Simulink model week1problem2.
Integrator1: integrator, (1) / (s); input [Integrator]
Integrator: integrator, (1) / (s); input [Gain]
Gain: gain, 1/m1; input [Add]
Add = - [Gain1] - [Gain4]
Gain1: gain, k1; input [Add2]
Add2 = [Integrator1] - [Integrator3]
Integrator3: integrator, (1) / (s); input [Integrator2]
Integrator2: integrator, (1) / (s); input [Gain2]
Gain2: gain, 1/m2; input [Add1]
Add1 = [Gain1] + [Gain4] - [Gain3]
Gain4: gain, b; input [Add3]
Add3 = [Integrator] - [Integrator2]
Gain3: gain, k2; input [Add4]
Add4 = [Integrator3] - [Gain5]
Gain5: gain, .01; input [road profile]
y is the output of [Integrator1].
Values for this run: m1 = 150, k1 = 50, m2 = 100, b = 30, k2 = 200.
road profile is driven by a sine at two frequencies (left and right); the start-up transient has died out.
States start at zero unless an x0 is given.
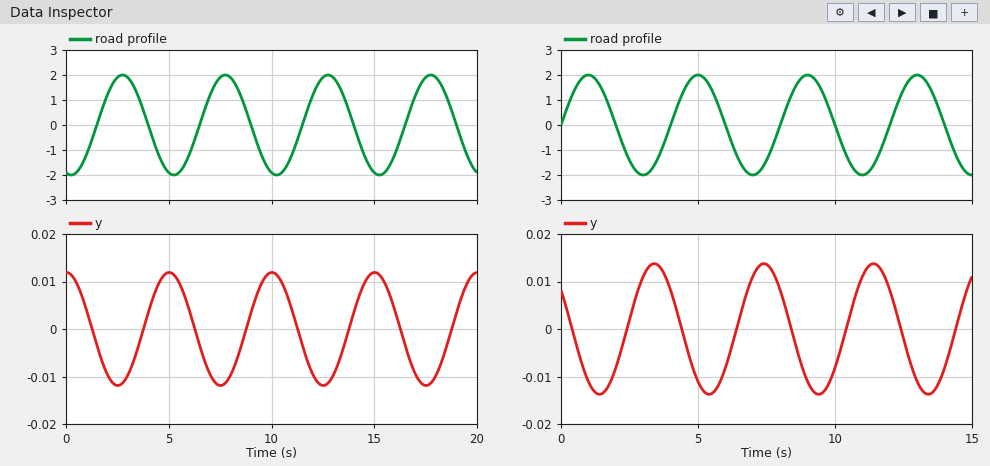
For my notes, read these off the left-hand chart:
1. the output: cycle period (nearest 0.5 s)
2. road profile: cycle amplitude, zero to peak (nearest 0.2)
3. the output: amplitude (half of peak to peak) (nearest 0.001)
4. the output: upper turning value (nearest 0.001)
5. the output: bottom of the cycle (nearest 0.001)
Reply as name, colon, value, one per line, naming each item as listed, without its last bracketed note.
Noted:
the output: cycle period: 5.0 s
road profile: cycle amplitude, zero to peak: 2.0
the output: amplitude (half of peak to peak): 0.012
the output: upper turning value: 0.012
the output: bottom of the cycle: -0.012
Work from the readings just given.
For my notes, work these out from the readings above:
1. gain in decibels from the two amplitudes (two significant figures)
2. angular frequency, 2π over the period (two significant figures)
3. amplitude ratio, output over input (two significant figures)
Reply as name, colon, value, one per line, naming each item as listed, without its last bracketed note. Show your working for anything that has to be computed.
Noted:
gain in decibels from the two amplitudes: 20 log10(0.012 / 2) = -44 dB
angular frequency, 2π over the period: 2π / 5 = 1.3 rad/s
amplitude ratio, output over input: 0.012 / 2 = 0.0060
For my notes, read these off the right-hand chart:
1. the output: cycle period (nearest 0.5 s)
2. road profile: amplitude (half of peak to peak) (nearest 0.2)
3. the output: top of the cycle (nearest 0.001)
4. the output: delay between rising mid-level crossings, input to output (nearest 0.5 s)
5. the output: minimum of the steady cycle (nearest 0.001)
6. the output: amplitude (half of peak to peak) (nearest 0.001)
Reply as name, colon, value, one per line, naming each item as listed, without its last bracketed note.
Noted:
the output: cycle period: 4.0 s
road profile: amplitude (half of peak to peak): 2.0
the output: top of the cycle: 0.014
the output: delay between rising mid-level crossings, input to output: 2.5 s
the output: minimum of the steady cycle: -0.014
the output: amplitude (half of peak to peak): 0.014
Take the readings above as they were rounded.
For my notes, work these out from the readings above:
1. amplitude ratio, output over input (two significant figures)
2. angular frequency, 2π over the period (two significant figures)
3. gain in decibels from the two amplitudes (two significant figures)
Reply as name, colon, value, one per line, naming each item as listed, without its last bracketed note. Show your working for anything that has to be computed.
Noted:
amplitude ratio, output over input: 0.014 / 2 = 0.0070
angular frequency, 2π over the period: 2π / 4 = 1.6 rad/s
gain in decibels from the two amplitudes: 20 log10(0.014 / 2) = -43 dB
